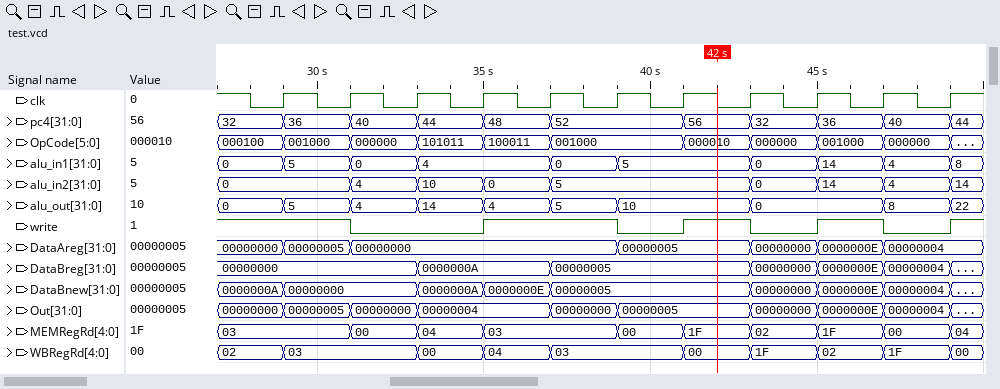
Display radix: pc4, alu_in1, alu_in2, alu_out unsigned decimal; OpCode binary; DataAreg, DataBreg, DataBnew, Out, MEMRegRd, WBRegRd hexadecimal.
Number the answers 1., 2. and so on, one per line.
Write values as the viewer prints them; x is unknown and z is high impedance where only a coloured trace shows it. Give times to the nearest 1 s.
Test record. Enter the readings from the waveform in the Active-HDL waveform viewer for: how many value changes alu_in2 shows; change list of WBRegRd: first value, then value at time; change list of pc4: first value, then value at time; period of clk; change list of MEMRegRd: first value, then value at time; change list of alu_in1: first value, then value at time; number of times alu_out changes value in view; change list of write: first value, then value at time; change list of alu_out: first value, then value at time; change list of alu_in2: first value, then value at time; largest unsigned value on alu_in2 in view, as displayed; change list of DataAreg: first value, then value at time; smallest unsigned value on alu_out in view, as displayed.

1. 8
2. 02, 03 at 29 s, 00 at 33 s, 04 at 35 s, 03 at 37 s, 00 at 41 s, 1F at 43 s, 02 at 45 s, 1F at 47 s, 00 at 49 s
3. 32, 36 at 29 s, 40 at 31 s, 44 at 33 s, 48 at 35 s, 52 at 37 s, 56 at 41 s, 32 at 43 s, 36 at 45 s, 40 at 47 s, 44 at 49 s
4. 2 s
5. 03, 00 at 31 s, 04 at 33 s, 03 at 35 s, 00 at 39 s, 1F at 41 s, 02 at 43 s, 1F at 45 s, 00 at 47 s, 04 at 49 s
6. 0, 5 at 29 s, 0 at 31 s, 4 at 33 s, 0 at 37 s, 5 at 39 s, 0 at 43 s, 14 at 45 s, 4 at 47 s, 8 at 49 s
7. 9
8. 1, 0 at 31 s, 1 at 35 s, 0 at 39 s, 1 at 41 s, 0 at 43 s, 1 at 45 s, 0 at 47 s, 1 at 49 s
9. 0, 5 at 29 s, 4 at 31 s, 14 at 33 s, 4 at 35 s, 5 at 37 s, 10 at 39 s, 0 at 43 s, 8 at 47 s, 22 at 49 s
10. 0, 4 at 31 s, 10 at 33 s, 0 at 35 s, 5 at 37 s, 0 at 43 s, 14 at 45 s, 4 at 47 s, 14 at 49 s
11. 14
12. 00000000, 00000005 at 29 s, 00000000 at 31 s, 00000005 at 39 s, 00000000 at 43 s, 0000000E at 45 s, 00000004 at 47 s
13. 0
